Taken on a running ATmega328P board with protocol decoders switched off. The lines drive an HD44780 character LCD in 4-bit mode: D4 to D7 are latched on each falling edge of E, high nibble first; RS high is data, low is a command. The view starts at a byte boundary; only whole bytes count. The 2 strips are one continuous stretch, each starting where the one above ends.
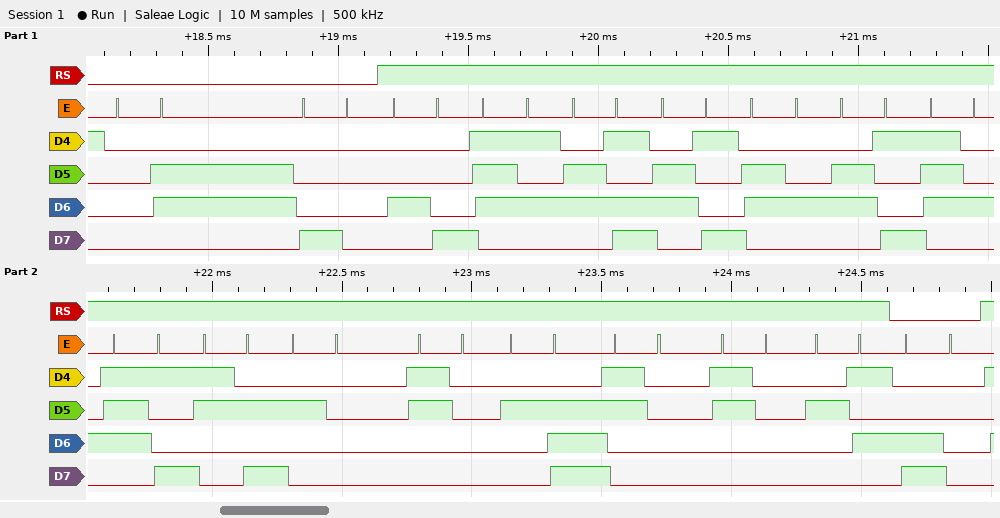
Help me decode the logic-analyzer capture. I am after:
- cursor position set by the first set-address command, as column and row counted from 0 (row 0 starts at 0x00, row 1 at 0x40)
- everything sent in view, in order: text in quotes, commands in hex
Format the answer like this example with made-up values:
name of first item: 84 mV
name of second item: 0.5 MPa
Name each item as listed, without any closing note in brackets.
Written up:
cursor position set by the first set-address command, as column and row counted from 0: column 0, row 0
everything sent in view, in order: text in quotes, commands in hex: 0x06 0x80 "Humidity: 0.00%" 0xC0
